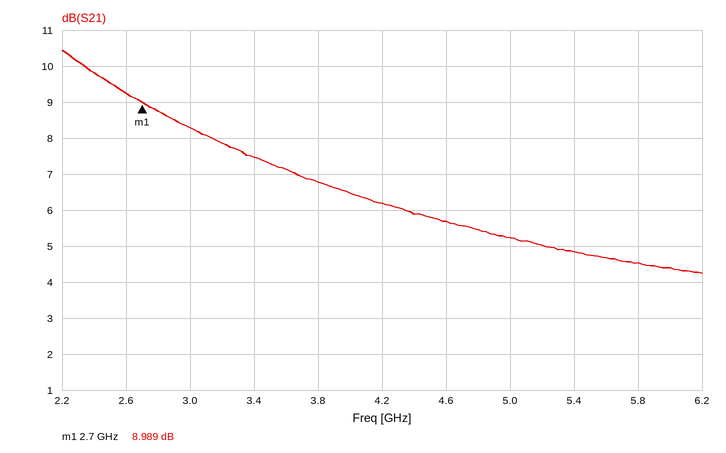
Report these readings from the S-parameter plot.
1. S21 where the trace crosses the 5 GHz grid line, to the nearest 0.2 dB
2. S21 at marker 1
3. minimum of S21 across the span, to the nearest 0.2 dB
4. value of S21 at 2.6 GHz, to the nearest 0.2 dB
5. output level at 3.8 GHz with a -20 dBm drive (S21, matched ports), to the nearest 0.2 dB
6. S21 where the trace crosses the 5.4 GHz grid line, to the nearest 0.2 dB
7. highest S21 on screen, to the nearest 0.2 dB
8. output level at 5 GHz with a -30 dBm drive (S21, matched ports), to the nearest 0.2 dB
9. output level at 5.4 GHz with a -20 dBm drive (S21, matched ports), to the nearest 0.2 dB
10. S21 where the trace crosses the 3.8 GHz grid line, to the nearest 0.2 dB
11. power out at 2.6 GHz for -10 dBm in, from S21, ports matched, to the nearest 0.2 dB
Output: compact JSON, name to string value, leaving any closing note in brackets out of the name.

{"S21 where the trace crosses the 5 GHz grid line, to the nearest 0.2 dB": "5.2 dB", "S21 at marker 1": "8.989 dB", "minimum of S21 across the span, to the nearest 0.2 dB": "4.2 dB", "value of S21 at 2.6 GHz, to the nearest 0.2 dB": "9.2 dB", "output level at 3.8 GHz with a -20 dBm drive (S21, matched ports), to the nearest 0.2 dB": "-13.2 dBm", "S21 where the trace crosses the 5.4 GHz grid line, to the nearest 0.2 dB": "4.8 dB", "highest S21 on screen, to the nearest 0.2 dB": "10.4 dB", "output level at 5 GHz with a -30 dBm drive (S21, matched ports), to the nearest 0.2 dB": "-24.8 dBm", "output level at 5.4 GHz with a -20 dBm drive (S21, matched ports), to the nearest 0.2 dB": "-15.2 dBm", "S21 where the trace crosses the 3.8 GHz grid line, to the nearest 0.2 dB": "6.8 dB", "power out at 2.6 GHz for -10 dBm in, from S21, ports matched, to the nearest 0.2 dB": "-0.8 dBm"}
